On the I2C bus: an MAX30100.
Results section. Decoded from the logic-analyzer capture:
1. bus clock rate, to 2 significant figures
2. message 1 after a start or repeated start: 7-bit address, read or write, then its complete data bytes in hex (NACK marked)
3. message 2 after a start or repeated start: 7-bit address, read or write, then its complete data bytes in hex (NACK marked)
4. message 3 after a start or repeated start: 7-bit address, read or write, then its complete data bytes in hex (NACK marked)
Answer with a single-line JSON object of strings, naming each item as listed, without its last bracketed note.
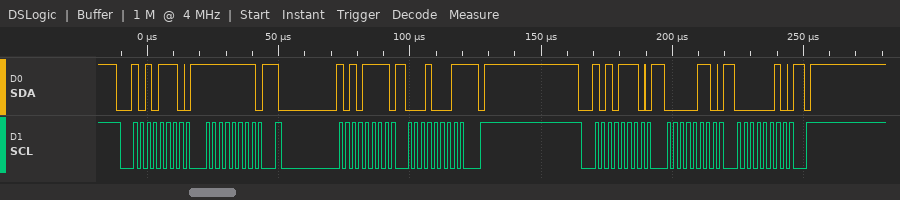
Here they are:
{"bus clock rate, to 2 significant figures": "400 kHz", "message 1 after a start or repeated start: 7-bit address, read or write, then its complete data bytes in hex": "0x57 write: FF", "message 2 after a start or repeated start: 7-bit address, read or write, then its complete data bytes in hex": "0x57 read: 11 NACK", "message 3 after a start or repeated start: 7-bit address, read or write, then its complete data bytes in hex": "0x57 write: 06 02"}
